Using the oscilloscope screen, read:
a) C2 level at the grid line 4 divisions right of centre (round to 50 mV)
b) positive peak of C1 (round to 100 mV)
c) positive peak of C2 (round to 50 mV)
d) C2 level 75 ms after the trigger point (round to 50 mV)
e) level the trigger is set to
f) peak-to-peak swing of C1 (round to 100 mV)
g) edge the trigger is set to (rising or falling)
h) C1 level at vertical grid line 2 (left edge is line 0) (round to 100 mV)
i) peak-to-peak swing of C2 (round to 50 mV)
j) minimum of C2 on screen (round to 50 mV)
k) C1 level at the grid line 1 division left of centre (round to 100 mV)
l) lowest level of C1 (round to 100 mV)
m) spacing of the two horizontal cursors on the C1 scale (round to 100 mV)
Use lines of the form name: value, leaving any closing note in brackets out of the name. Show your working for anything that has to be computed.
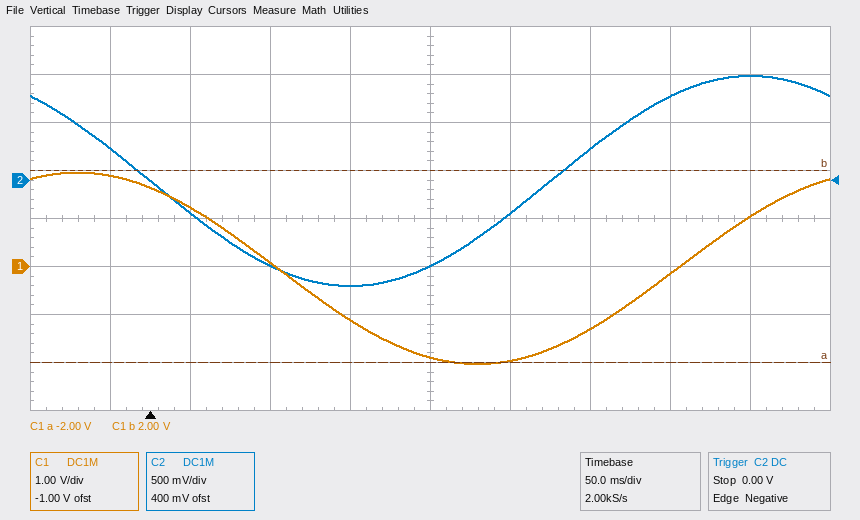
C2 level at the grid line 4 divisions right of centre: 1.10 V
positive peak of C1: 2.0 V
positive peak of C2: 1.10 V
C2 level 75 ms after the trigger point: -900 mV
level the trigger is set to: 0.00 V
peak-to-peak swing of C1: 2.0 V − (-2.0 V) = 4.0 V
edge the trigger is set to: falling
C1 level at vertical grid line 2 (left edge is line 0): 1.2 V
peak-to-peak swing of C2: 1.10 V − (-1.10 V) = 2.20 V
minimum of C2 on screen: -1.10 V
C1 level at the grid line 1 division left of centre: -1.1 V
lowest level of C1: -2.0 V
spacing of the two horizontal cursors on the C1 scale: 4.0 V
